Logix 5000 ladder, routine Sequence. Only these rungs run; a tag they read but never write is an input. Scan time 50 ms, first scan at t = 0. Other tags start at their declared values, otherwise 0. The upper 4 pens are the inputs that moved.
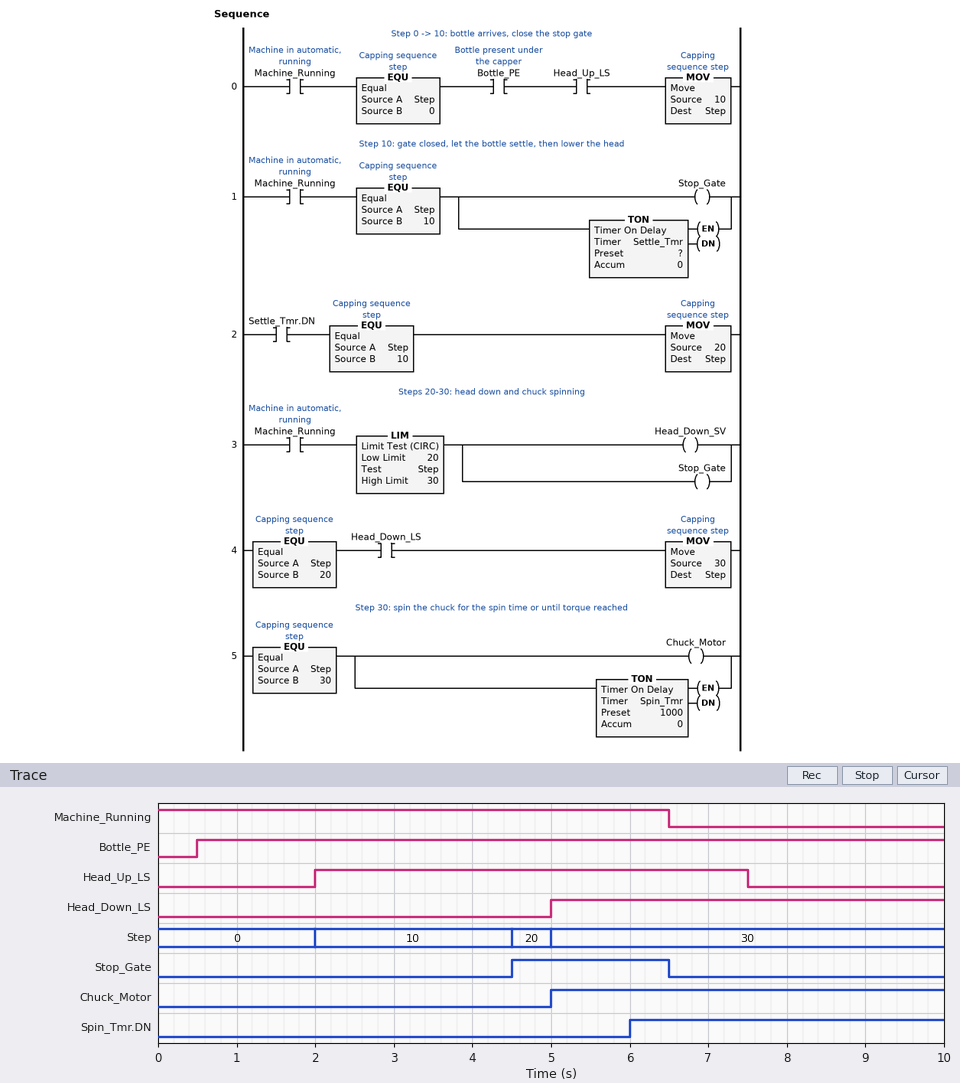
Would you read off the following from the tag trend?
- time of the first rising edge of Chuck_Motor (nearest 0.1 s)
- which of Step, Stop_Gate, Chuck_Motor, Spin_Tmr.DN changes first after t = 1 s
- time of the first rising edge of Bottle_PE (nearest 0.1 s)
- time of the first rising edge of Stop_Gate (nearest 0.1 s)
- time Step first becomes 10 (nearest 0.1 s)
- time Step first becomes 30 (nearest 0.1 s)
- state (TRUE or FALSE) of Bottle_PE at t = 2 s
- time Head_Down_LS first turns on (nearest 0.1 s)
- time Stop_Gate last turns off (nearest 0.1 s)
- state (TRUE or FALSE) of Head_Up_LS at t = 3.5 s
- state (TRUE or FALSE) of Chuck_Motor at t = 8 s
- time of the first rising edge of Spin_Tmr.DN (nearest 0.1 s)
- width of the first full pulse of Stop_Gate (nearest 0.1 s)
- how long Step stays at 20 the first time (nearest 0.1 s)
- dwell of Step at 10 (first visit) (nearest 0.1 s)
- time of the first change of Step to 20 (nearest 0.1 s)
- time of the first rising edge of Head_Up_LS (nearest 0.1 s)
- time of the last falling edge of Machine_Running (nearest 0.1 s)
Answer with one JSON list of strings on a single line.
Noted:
["5.0 s", "Step", "0.5 s", "4.5 s", "2.0 s", "5.0 s", "TRUE", "5.0 s", "6.5 s", "TRUE", "TRUE", "6.0 s", "2.0 s", "0.5 s", "2.5 s", "4.5 s", "2.0 s", "6.5 s"]
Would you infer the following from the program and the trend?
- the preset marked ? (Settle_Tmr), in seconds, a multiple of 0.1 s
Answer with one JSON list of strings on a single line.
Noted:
["2.5 s"]
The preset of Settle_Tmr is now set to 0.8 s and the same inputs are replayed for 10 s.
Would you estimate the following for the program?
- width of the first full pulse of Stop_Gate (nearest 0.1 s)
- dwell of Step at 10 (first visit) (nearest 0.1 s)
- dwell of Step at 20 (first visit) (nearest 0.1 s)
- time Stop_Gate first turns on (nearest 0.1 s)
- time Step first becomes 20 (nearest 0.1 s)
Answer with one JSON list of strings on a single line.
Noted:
["3.7 s", "0.8 s", "2.2 s", "2.8 s", "2.8 s"]
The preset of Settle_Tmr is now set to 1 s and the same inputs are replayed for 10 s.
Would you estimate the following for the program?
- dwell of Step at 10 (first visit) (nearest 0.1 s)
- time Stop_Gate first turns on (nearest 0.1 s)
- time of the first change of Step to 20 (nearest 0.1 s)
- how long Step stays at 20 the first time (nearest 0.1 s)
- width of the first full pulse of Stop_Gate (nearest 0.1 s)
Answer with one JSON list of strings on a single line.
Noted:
["1.0 s", "3.0 s", "3.0 s", "2.0 s", "3.5 s"]
